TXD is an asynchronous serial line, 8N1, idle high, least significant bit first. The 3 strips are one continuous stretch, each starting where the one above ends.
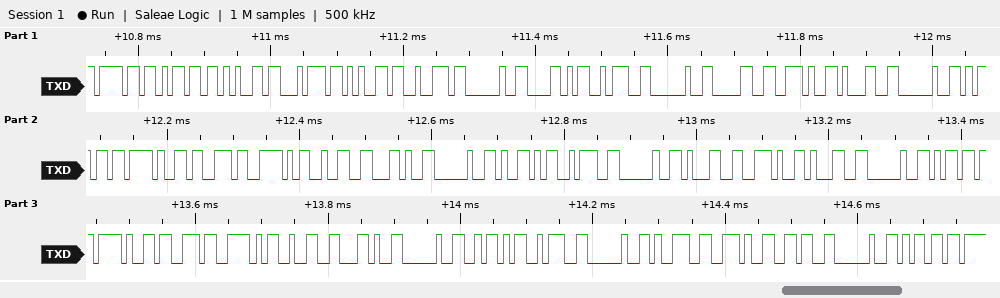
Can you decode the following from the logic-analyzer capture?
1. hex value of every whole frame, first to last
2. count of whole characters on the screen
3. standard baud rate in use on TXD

6F 6D 65 74 65 72 20 58 3A 20 30 2E 31 20 6D 2F 73 5E 32 2C 20 59 3A 20 31 2E 31 20 6D 2F 73 5E 32 2C 20 5A 3A 20 39 2E 36 20 6D
43
115200 baud
